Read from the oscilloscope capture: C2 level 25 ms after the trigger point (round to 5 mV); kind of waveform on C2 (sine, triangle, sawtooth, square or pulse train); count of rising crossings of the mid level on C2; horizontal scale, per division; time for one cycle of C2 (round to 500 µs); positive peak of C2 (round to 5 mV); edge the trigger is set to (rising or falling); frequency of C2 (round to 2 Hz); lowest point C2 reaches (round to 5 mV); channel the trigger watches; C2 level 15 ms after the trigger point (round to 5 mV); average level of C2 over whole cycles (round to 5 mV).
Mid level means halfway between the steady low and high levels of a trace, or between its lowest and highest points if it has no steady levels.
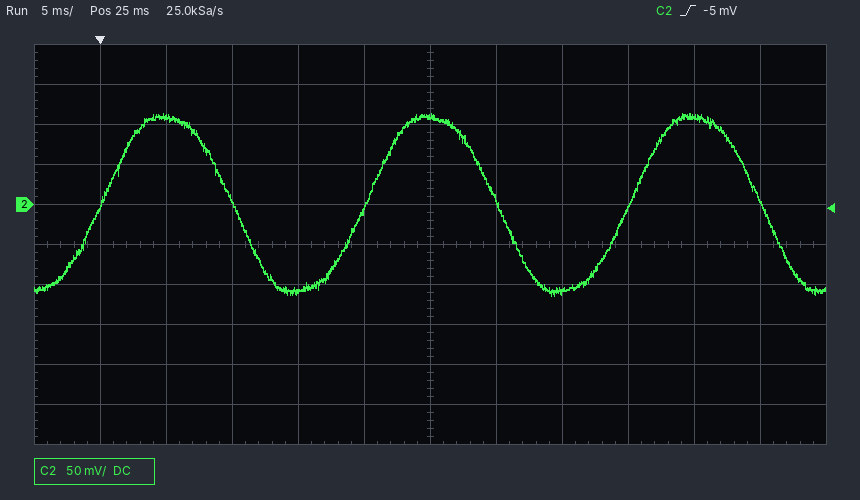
110 mV
sine
3
5 ms
20.0 ms
115 mV
rising
50 Hz
-115 mV
C2
-110 mV
0 mV
